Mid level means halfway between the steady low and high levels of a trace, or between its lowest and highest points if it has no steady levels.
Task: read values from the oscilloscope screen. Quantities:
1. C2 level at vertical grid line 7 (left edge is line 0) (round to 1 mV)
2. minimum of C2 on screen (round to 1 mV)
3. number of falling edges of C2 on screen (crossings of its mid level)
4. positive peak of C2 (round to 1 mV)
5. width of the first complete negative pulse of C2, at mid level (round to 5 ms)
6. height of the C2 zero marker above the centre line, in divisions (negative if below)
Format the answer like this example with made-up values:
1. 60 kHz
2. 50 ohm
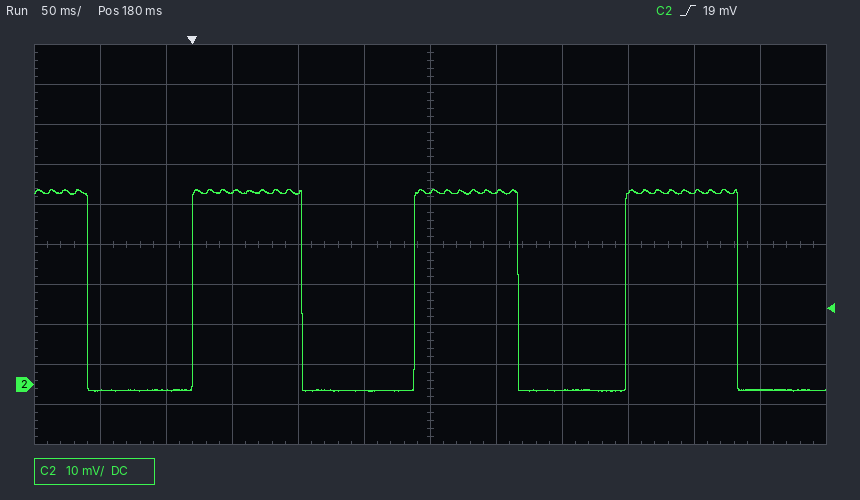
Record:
1. 48 mV
2. -2 mV
3. 4
4. 49 mV
5. 80 ms
6. -3.5 div
